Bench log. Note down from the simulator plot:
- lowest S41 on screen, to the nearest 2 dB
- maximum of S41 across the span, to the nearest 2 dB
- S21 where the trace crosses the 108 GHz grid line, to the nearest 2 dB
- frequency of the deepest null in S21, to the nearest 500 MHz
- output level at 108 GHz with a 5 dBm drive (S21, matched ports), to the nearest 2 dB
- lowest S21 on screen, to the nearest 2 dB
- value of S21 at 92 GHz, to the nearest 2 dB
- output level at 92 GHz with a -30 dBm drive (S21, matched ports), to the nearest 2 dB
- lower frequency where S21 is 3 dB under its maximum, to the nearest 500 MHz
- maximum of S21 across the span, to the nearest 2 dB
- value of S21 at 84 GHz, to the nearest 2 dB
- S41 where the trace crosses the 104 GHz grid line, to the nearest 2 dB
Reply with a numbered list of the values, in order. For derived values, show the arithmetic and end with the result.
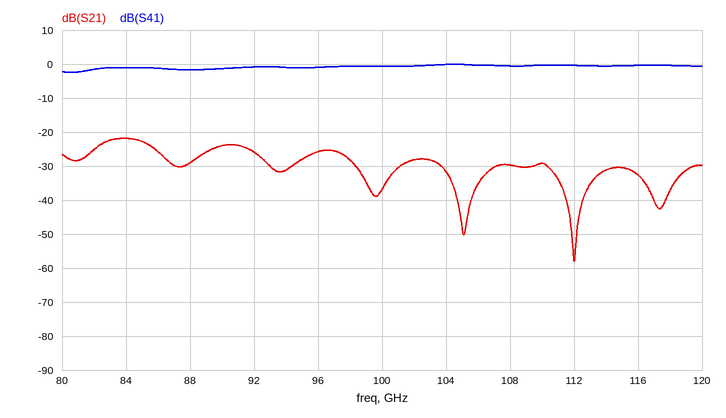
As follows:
1. -2 dB
2. 0 dB
3. -30 dB
4. 112.0 GHz
5. 5 dBm + (-30 dB) = -24 dBm
6. -58 dB
7. -26 dB
8. -30 dBm + (-26 dB) = -56 dBm
9. 82.0 GHz
10. -22 dB
11. -22 dB
12. 0 dB
